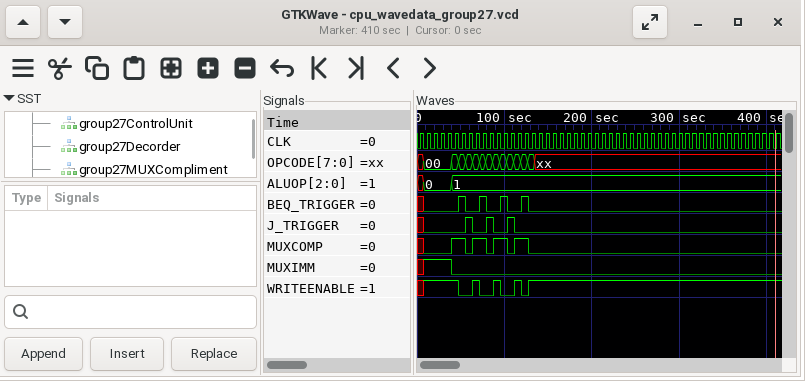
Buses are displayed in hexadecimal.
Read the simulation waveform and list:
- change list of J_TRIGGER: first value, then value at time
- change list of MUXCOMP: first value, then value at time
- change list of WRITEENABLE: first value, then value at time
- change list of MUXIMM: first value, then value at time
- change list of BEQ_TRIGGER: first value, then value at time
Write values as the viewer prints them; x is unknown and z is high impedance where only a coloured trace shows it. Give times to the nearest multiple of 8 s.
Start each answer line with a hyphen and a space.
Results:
- x, 0 at 8 s, 1 at 56 s, 0 at 64 s, 1 at 80 s, 0 at 88 s, 1 at 104 s, 0 at 112 s
- x, 0 at 8 s, 1 at 40 s, 0 at 56 s, 1 at 64 s, 0 at 80 s, 1 at 88 s, 0 at 104 s, 1 at 112 s, 0 at 128 s
- x, 1 at 8 s, 0 at 48 s, 1 at 64 s, 0 at 72 s, 1 at 88 s, 0 at 96 s, 1 at 112 s, 0 at 120 s, 1 at 128 s
- x, 1 at 8 s, 0 at 40 s
- x, 0 at 8 s, 1 at 48 s, 0 at 56 s, 1 at 72 s, 0 at 80 s, 1 at 96 s, 0 at 104 s, 1 at 120 s, 0 at 128 s
